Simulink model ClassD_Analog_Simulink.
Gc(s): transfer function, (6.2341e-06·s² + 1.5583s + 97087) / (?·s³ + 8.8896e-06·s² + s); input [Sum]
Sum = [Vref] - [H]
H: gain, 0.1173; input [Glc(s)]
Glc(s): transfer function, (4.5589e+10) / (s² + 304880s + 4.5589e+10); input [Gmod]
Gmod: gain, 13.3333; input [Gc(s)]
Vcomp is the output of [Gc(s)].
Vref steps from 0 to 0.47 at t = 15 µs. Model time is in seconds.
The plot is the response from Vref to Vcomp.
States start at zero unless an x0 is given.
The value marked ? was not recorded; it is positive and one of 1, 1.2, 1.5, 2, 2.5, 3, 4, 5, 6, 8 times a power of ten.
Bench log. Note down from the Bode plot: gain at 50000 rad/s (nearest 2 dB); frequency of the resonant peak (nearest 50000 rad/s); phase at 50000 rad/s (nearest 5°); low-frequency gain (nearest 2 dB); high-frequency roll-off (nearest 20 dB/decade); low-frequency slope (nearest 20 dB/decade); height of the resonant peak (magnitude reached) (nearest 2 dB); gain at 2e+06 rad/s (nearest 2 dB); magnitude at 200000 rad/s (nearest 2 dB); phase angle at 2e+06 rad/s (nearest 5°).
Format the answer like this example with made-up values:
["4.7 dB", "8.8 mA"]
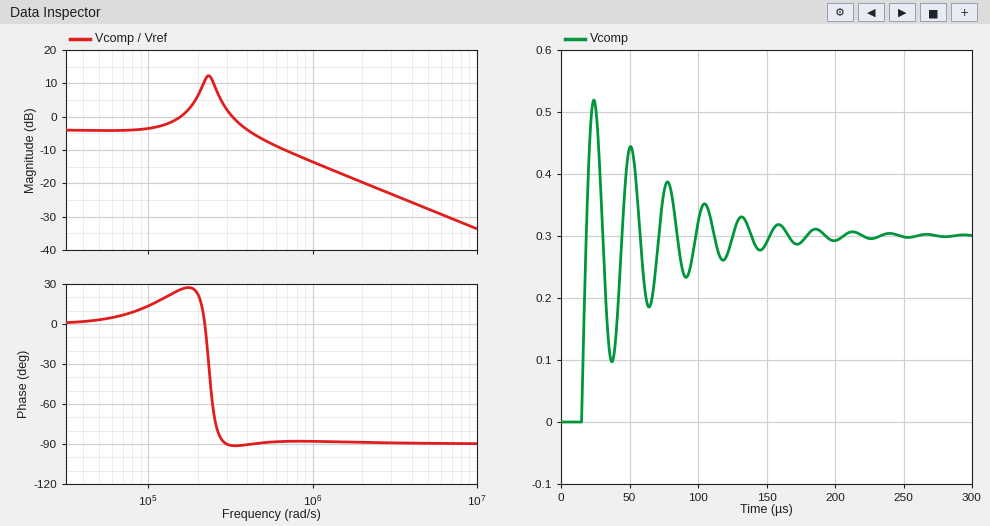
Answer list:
["-4 dB", "250000 rad/s", "5°", "-4 dB", "-20 dB/decade", "0 dB/decade", "12 dB", "-20 dB", "6 dB", "-90°"]
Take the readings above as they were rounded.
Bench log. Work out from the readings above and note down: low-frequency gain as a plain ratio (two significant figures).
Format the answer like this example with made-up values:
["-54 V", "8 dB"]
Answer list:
["0.63"]
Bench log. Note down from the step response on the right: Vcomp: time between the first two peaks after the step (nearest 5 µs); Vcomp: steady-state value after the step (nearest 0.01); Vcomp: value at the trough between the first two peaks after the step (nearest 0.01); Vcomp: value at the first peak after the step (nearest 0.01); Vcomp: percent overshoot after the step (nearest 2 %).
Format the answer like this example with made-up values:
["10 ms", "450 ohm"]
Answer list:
["25 µs", "0.30", "0.10", "0.52", "72 %"]
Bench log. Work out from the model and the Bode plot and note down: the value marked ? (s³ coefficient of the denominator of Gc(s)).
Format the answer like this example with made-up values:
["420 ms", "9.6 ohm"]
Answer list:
["3e-11"]
